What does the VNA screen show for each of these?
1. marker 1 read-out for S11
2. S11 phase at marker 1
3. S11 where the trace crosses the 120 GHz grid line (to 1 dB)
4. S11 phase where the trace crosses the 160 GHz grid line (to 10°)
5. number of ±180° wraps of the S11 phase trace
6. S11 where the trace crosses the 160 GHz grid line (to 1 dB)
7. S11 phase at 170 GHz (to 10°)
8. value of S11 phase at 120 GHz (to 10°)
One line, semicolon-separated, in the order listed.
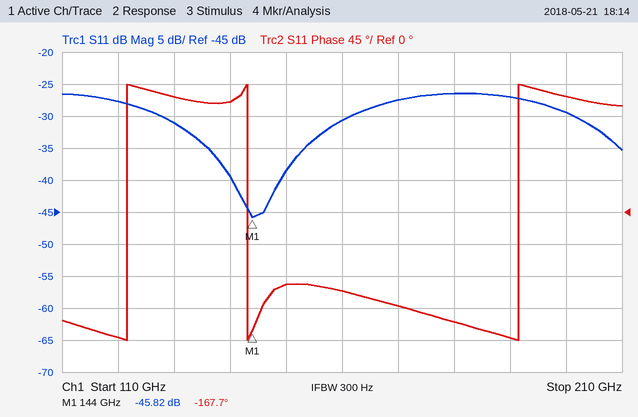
-45.82 dB; -167.7°; -28 dB; -110°; 3; -31 dB; -130°; -180°
